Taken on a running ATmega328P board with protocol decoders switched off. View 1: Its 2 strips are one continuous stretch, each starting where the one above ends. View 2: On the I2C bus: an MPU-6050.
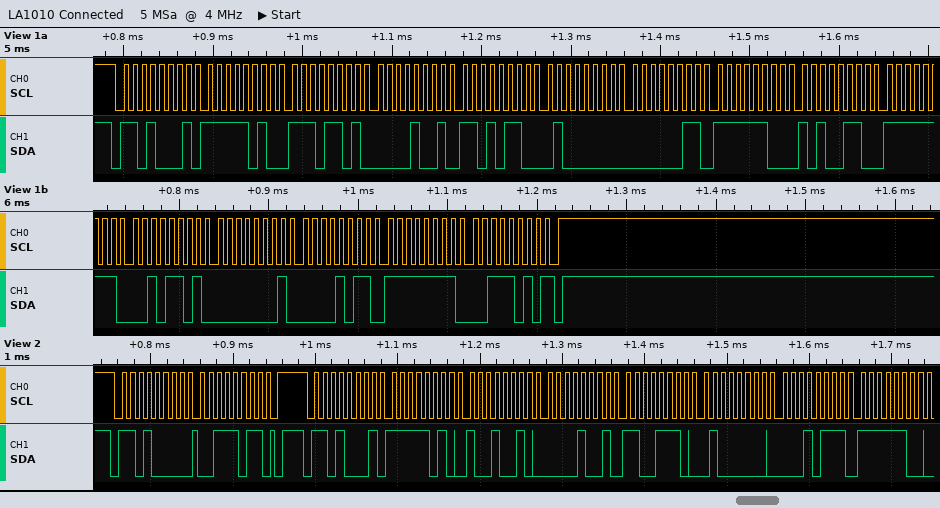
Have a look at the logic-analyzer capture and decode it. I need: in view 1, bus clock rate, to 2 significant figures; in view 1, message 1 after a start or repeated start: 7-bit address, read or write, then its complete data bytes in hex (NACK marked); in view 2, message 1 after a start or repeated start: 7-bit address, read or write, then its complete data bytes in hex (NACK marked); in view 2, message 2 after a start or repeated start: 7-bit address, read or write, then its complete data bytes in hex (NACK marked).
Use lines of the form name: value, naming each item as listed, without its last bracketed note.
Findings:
in view 1, bus clock rate, to 2 significant figures: 100 kHz
in view 1, message 1 after a start or repeated start: 7-bit address, read or write, then its complete data bytes in hex: 0x68 read: FA ED 09 D6 40 03 FC A6 FF 2D 01 0B FF 3A NACK
in view 2, message 1 after a start or repeated start: 7-bit address, read or write, then its complete data bytes in hex: 0x68 write: 3B
in view 2, message 2 after a start or repeated start: 7-bit address, read or write, then its complete data bytes in hex: 0x68 read: FA 92 09 CE 40 17 FC
